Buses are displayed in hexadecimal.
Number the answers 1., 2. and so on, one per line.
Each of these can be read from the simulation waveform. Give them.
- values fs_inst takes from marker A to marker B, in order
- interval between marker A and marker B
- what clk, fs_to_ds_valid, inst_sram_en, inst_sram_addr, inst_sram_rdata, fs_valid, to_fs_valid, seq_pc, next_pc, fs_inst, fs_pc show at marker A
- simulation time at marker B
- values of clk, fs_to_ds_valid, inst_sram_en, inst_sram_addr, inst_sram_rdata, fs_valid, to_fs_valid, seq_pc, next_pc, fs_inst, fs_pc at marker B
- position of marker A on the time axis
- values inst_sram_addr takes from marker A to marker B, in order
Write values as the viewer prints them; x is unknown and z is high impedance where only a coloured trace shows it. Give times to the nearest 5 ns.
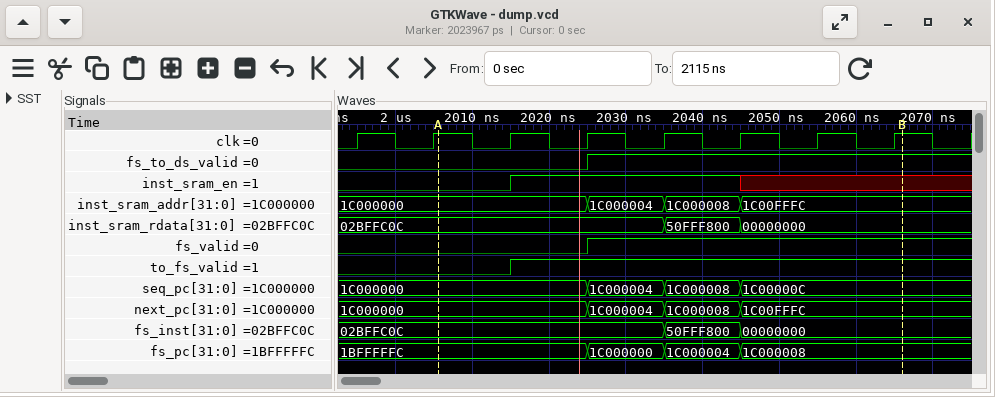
1. 02BFFC0C, 50FFF800, 00000000
2. 60 ns
3. clk=1, fs_to_ds_valid=0, inst_sram_en=0, inst_sram_addr=1C000000, inst_sram_rdata=02BFFC0C, fs_valid=0, to_fs_valid=0, seq_pc=1C000000, next_pc=1C000000, fs_inst=02BFFC0C, fs_pc=1BFFFFFC
4. 2065 ns
5. clk=1, fs_to_ds_valid=1, inst_sram_en=x, inst_sram_addr=1C00FFFC, inst_sram_rdata=00000000, fs_valid=1, to_fs_valid=1, seq_pc=1C00000C, next_pc=1C00FFFC, fs_inst=00000000, fs_pc=1C000008
6. 2005 ns
7. 1C000000, 1C000004, 1C000008, 1C00FFFC
